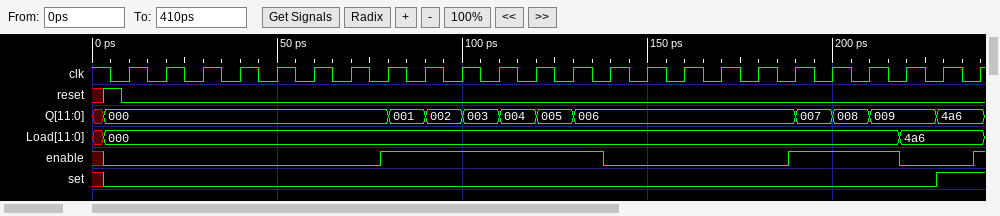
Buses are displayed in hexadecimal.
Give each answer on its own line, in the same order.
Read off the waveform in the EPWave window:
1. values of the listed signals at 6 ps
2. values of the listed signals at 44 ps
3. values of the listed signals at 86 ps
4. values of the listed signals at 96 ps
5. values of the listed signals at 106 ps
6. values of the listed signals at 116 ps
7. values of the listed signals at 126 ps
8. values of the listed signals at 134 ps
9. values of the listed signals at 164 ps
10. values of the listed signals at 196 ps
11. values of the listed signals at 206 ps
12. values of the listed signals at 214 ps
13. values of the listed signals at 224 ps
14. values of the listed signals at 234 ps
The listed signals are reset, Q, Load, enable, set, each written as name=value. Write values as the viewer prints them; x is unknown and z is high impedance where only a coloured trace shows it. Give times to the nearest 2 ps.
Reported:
reset=1, Q=000, Load=000, enable=0, set=0
reset=0, Q=000, Load=000, enable=0, set=0
reset=0, Q=001, Load=000, enable=1, set=0
reset=0, Q=002, Load=000, enable=1, set=0
reset=0, Q=003, Load=000, enable=1, set=0
reset=0, Q=004, Load=000, enable=1, set=0
reset=0, Q=005, Load=000, enable=1, set=0
reset=0, Q=006, Load=000, enable=1, set=0
reset=0, Q=006, Load=000, enable=0, set=0
reset=0, Q=007, Load=000, enable=1, set=0
reset=0, Q=008, Load=000, enable=1, set=0
reset=0, Q=009, Load=000, enable=1, set=0
reset=0, Q=009, Load=4a6, enable=0, set=0
reset=0, Q=4a6, Load=4a6, enable=0, set=1
